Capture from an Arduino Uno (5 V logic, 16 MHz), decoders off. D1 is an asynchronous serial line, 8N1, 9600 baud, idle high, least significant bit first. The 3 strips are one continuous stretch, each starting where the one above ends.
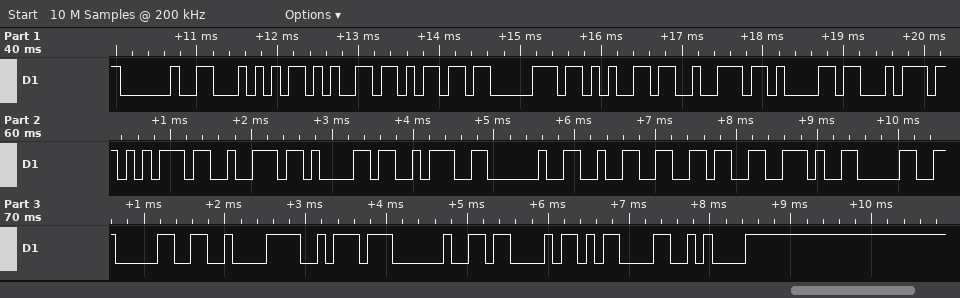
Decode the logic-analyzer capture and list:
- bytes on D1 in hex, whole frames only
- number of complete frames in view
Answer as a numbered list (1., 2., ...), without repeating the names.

1. 20 54 65 6D 70 65 72 61 74 75 72 61 3A 20 32 36 2E 30 30 C2 BA 20 43 0D 0A
2. 25
